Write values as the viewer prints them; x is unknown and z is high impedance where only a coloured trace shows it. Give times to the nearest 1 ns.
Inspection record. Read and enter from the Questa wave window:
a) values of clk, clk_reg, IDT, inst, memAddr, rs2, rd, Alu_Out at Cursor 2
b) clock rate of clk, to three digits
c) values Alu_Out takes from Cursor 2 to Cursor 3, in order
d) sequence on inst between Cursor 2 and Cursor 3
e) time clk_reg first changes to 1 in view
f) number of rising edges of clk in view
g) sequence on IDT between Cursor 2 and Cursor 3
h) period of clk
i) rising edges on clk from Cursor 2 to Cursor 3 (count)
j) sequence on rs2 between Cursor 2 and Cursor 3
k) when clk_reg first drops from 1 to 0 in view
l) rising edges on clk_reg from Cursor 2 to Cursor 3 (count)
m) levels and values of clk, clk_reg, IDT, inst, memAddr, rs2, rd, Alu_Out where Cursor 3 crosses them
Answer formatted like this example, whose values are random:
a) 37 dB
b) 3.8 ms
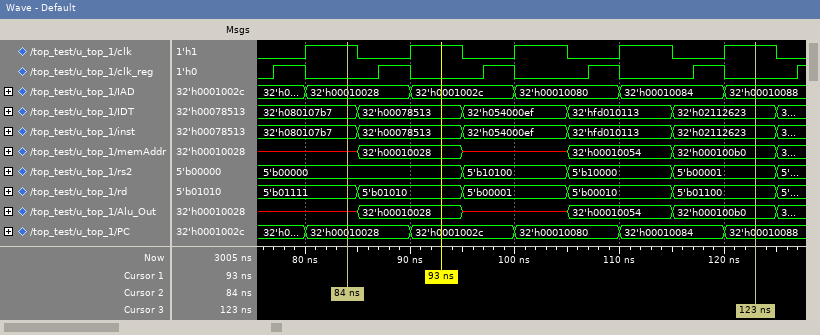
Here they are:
a) clk=1, clk_reg=0, IDT=32'h080107b7, inst=32'h080107b7, memAddr=x, rs2=5'b00000, rd=5'b01111, Alu_Out=x
b) 100 MHz
c) x, 32'h00010028, x, 32'h00010054, 32'h000100b0
d) 32'h080107b7, 32'h00078513, 32'h054000ef, 32'hfd010113, 32'h02112623
e) 77 ns
f) 5
g) 32'h080107b7, 32'h00078513, 32'h054000ef, 32'hfd010113, 32'h02112623
h) 10 ns
i) 4
j) 5'b00000, 5'b10100, 5'b10000, 5'b00001
k) 80 ns
l) 4
m) clk=1, clk_reg=0, IDT=32'h02112623, inst=32'h02112623, memAddr=32'h000100b0, rs2=5'b00001, rd=5'b01100, Alu_Out=32'h000100b0
